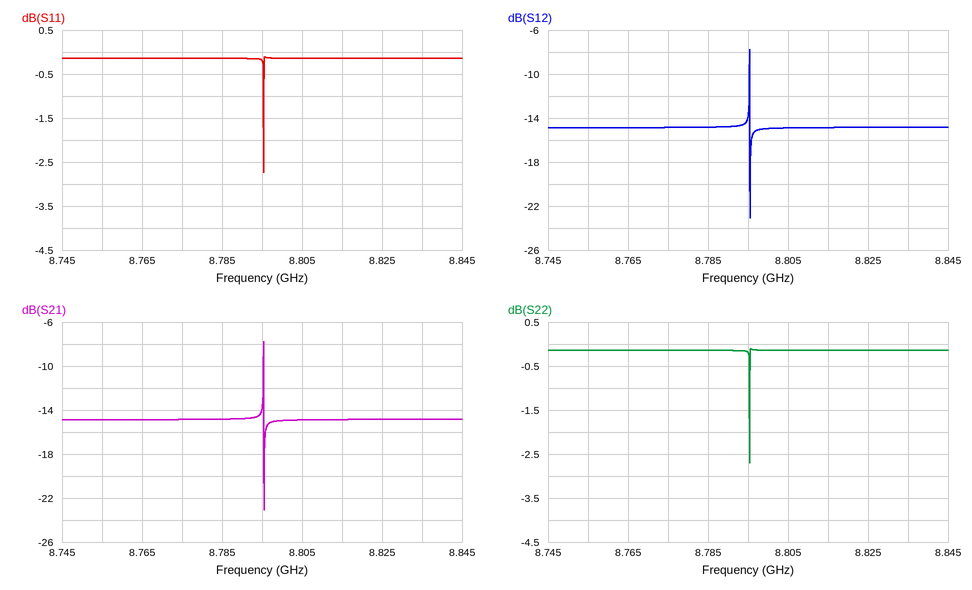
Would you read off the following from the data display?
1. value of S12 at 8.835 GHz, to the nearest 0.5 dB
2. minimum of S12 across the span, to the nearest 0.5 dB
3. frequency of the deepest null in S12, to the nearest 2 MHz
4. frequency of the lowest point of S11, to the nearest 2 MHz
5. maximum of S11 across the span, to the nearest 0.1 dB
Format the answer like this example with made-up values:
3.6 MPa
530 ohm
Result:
-15.0 dB
-23.0 dB
8.796 GHz
8.796 GHz
-0.1 dB
